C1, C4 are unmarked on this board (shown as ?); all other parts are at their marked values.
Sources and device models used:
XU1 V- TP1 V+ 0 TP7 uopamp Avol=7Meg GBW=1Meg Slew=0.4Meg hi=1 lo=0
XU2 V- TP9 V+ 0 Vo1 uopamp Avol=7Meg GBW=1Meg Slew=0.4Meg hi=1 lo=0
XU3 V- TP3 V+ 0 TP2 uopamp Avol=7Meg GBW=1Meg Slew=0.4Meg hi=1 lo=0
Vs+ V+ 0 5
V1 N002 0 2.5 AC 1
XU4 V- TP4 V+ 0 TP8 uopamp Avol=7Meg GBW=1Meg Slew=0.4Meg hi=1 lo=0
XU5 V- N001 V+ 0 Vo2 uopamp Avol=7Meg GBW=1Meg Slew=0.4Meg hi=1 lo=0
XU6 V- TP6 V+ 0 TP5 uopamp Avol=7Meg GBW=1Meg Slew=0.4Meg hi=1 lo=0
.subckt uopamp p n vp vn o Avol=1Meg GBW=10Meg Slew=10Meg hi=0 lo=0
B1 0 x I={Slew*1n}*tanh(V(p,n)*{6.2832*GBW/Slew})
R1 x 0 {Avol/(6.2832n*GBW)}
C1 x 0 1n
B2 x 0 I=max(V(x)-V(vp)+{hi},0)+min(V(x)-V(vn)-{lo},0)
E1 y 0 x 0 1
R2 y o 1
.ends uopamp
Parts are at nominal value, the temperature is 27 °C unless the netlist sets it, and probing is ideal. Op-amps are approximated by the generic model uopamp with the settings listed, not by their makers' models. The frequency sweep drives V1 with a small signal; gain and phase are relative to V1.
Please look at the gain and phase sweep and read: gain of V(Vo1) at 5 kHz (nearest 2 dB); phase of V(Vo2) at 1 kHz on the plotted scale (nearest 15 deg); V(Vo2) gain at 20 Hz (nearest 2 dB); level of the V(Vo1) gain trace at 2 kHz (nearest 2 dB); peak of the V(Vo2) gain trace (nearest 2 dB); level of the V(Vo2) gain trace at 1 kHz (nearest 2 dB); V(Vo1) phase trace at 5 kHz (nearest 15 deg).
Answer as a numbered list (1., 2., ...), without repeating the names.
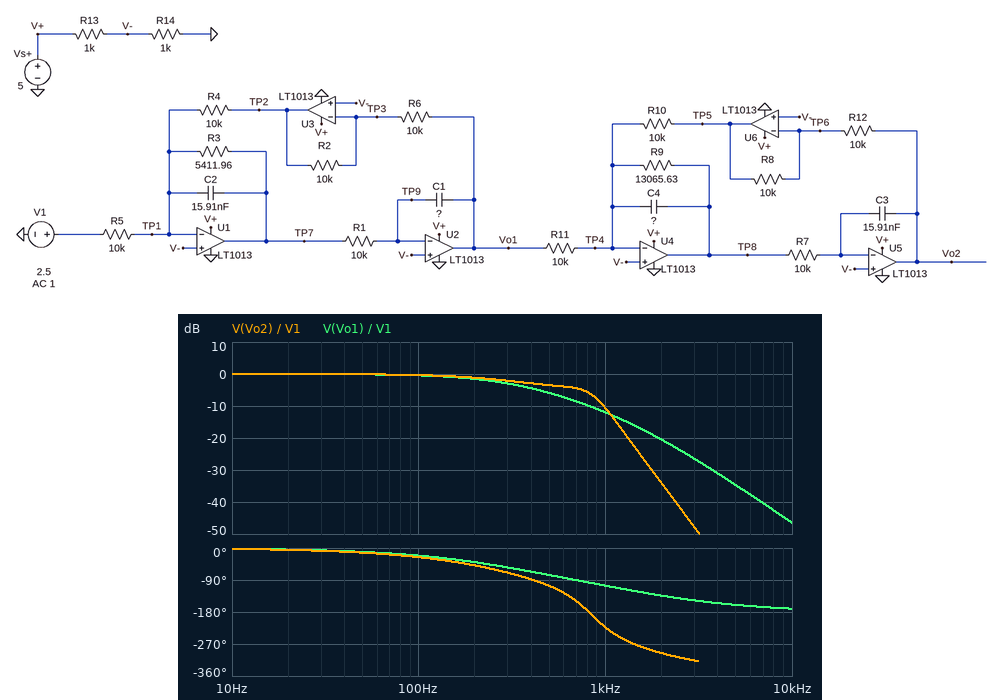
1. -34 dB
2. -225 deg
3. 0 dB
4. -20 dB
5. 0 dB
6. -10 dB
7. -165 deg
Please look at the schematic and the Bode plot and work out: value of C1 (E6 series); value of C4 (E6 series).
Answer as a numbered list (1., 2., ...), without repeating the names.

1. 33 nF
2. 22 nF
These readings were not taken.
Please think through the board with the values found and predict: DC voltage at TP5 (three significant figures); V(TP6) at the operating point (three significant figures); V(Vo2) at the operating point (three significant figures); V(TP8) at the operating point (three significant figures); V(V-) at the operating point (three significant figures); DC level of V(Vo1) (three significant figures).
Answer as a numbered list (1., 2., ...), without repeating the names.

1. 2.50 V
2. 2.50 V
3. 2.50 V
4. 2.50 V
5. 2.50 V
6. 2.50 V
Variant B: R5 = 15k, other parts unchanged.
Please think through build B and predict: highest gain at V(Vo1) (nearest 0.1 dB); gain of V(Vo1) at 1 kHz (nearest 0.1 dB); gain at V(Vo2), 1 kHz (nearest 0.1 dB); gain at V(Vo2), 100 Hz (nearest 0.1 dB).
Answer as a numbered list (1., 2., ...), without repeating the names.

1. -3.5 dB
2. -15.5 dB
3. -14.1 dB
4. -3.9 dB
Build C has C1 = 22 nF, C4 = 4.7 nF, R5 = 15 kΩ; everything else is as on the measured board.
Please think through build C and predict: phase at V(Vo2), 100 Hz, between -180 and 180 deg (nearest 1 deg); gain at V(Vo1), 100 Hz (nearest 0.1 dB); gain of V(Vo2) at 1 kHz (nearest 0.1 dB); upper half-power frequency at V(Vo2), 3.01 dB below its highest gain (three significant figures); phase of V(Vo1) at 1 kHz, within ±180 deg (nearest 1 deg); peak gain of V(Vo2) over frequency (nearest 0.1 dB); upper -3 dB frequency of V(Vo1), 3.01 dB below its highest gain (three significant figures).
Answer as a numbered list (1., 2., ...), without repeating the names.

1. -19 deg
2. -3.7 dB
3. -12.1 dB
4. 487 Hz
5. -99 deg
6. -3.5 dB
7. 488 Hz
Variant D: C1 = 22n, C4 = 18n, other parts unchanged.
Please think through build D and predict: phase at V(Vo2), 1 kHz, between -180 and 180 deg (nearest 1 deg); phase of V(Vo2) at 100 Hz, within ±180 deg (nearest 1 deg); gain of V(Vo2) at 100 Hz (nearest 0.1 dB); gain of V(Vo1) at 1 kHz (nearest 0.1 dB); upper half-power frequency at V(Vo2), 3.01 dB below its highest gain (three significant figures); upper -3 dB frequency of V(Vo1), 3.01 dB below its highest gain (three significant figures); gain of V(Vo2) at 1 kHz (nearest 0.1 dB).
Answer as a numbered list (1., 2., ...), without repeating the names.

1. 161 deg
2. -19 deg
3. -0.1 dB
4. -8.2 dB
5. 828 Hz
6. 488 Hz
7. -6.0 dB
